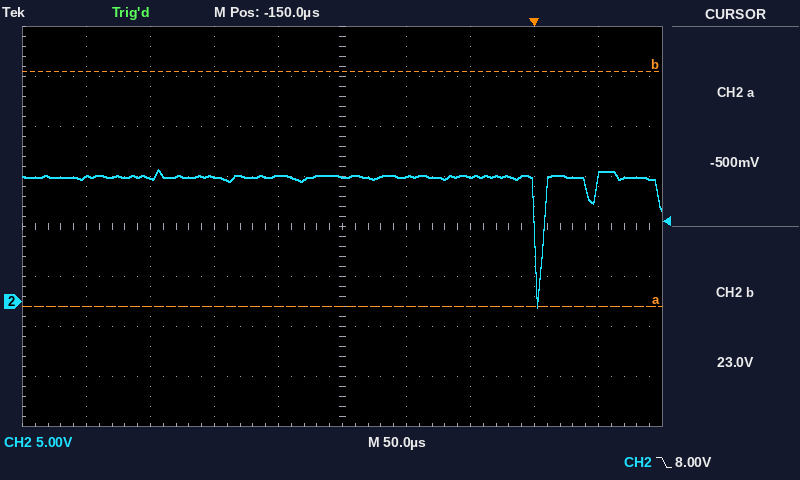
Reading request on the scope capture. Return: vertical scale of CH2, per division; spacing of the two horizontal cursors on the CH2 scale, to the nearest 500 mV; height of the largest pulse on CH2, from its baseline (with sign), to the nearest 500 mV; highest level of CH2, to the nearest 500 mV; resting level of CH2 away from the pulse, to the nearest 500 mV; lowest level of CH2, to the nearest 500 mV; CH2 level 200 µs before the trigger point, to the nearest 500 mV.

5 V
23.5 V
-13.0 V
13.0 V
12.5 V
-500 mV
12.5 V
